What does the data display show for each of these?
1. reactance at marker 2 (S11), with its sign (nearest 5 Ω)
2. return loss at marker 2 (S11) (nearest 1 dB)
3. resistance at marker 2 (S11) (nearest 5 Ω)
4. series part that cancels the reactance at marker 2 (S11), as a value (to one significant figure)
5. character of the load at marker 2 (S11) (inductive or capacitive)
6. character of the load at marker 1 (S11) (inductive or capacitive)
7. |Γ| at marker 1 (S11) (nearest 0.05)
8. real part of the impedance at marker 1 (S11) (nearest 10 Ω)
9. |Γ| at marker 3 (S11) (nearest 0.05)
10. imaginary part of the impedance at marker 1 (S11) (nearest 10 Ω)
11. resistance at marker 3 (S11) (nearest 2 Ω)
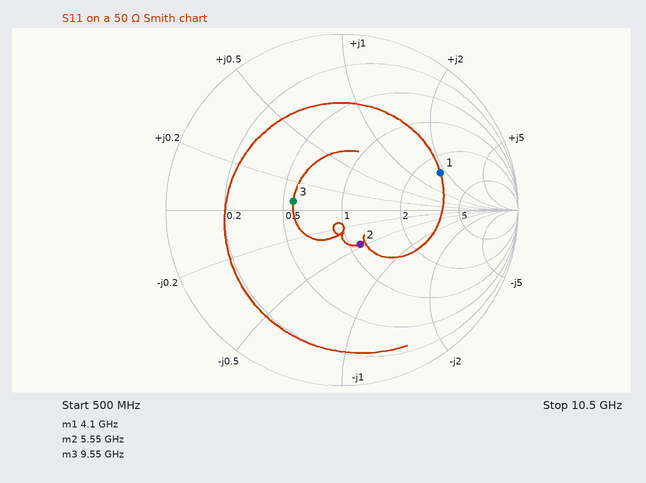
-25 Ω
13 dB
55 Ω
700 pH
capacitive
inductive
0.60
130 Ω
0.30
+90 Ω
28 Ω
